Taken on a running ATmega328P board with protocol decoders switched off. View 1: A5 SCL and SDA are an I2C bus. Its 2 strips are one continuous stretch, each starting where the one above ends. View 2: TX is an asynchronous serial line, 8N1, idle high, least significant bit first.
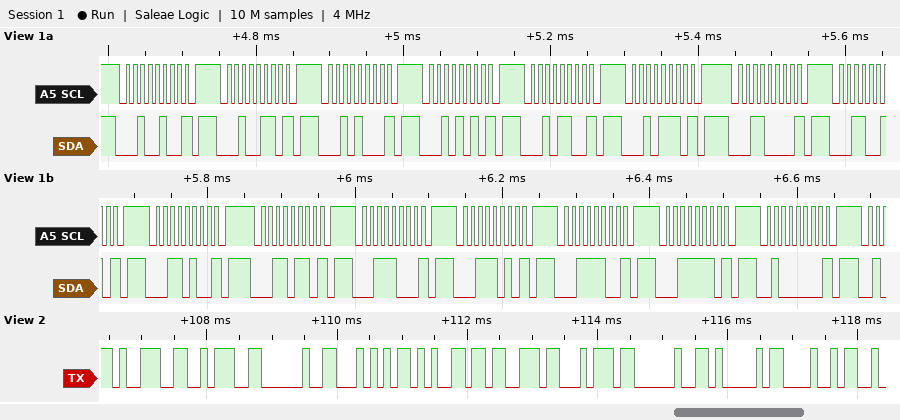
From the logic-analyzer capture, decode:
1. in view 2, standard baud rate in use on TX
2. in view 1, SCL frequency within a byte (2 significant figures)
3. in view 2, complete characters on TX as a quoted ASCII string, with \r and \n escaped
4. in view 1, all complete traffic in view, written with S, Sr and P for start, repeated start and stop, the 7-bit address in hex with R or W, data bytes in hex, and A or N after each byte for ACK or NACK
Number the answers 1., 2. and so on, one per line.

1. 9600 baud
2. 100 kHz
3. "9: Test AH"
4. S 12W N P S 13W N P S 14W N P S 15W N P S 16W N P S 17W N P S 18W N P S 19W N P S 1AW N P S 1BW N P S 1CW N P S 1DW N P S 1EW N P S 1FW N P S 20W N P
